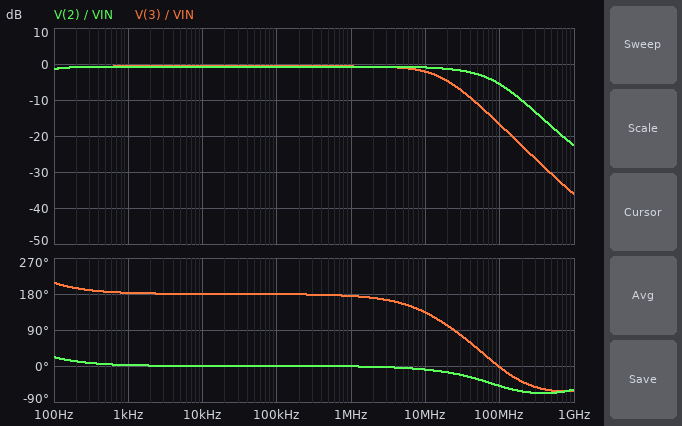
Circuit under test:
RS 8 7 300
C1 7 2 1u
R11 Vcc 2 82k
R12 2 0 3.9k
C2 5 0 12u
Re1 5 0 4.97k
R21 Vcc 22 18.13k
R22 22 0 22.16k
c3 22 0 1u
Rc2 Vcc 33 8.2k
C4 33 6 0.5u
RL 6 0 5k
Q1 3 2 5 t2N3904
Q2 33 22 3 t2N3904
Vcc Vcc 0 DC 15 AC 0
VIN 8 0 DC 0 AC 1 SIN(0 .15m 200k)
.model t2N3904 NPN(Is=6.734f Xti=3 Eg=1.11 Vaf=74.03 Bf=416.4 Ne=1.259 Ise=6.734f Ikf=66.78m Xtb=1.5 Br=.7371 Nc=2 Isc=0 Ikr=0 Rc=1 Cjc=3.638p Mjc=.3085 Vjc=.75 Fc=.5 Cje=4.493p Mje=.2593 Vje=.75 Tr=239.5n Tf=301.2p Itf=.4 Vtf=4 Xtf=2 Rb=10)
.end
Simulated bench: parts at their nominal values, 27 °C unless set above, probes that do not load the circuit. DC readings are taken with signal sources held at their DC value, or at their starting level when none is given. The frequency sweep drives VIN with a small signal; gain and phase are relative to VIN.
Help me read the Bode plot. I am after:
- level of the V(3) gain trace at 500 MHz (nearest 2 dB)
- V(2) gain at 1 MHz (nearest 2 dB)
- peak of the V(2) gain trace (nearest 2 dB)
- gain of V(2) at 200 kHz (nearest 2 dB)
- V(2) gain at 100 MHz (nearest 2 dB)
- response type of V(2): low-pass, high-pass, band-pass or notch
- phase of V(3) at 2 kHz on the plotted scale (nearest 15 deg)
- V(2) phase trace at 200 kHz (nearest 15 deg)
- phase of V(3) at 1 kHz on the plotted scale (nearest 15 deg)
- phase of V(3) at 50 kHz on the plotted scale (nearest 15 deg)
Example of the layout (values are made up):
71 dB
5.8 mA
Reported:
-30 dB
0 dB
0 dB
0 dB
-6 dB
low-pass
180 deg
0 deg
180 deg
180 deg
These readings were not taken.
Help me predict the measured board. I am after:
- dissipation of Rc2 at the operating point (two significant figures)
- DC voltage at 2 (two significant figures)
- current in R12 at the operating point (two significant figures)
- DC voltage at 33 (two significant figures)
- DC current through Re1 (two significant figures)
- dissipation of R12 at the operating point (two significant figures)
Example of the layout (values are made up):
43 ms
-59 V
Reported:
4.2 µW
680 mV
170 µA
15 V
23 µA
120 µW
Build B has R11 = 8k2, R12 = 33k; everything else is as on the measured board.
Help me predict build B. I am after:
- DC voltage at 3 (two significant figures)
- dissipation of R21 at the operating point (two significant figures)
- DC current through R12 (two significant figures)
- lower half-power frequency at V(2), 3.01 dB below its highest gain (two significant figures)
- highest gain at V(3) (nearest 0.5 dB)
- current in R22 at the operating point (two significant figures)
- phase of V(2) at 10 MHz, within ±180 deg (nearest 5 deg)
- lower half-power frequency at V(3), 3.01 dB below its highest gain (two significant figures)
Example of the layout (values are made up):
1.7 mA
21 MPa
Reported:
7.5 V
2.6 mW
250 µA
350 Hz
-24.5 dB
370 µA
-5 deg
6.4 Hz
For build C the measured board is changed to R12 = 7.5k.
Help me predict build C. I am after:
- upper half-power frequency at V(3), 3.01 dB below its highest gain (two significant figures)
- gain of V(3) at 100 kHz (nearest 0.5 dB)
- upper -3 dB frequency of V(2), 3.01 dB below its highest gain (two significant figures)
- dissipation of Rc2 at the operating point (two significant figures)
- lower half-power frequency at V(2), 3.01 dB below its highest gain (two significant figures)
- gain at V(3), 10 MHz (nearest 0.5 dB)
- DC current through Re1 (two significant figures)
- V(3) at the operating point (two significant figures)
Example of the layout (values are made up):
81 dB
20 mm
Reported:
39 MHz
-0.5 dB
46 MHz
130 µW
24 Hz
-0.5 dB
130 µA
7.6 V
